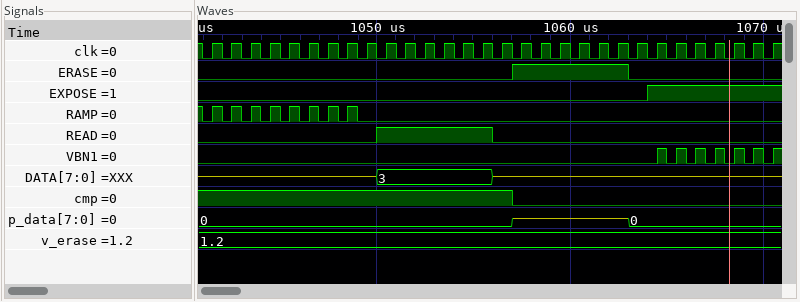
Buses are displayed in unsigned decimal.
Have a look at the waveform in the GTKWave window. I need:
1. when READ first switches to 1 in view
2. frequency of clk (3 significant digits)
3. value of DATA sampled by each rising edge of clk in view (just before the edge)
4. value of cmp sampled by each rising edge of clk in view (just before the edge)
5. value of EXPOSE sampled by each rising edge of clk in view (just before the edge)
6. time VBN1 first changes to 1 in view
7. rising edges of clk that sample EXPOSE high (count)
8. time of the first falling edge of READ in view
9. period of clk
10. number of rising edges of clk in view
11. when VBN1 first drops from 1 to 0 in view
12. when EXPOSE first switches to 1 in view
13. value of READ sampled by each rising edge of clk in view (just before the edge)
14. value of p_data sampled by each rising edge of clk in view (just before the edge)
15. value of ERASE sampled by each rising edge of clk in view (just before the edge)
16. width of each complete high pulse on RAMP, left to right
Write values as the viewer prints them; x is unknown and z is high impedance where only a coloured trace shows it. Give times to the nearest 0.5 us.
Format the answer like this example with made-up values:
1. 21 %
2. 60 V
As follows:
1. 1050 us
2. 1.00 MHz
3. z, z, z, z, z, z, z, z, z, 3, 3, 3, 3, 3, 3, z, z, z, z, z, z, z, z, z, z, z, z, z, z, z
4. 1 1 1 1 1 1 1 1 1 1 1 1 1 1 1 1 0 0 0 0 0 0 0 0 0 0 0 0 0 0
5. 0 0 0 0 0 0 0 0 0 0 0 0 0 0 0 0 0 0 0 0 0 0 0 1 1 1 1 1 1 1
6. 1064.5 us
7. 7
8. 1056 us
9. 1 us
10. 30
11. 1065 us
12. 1064 us
13. 0 0 0 0 0 0 0 0 0 1 1 1 1 1 1 0 0 0 0 0 0 0 0 0 0 0 0 0 0 0
14. 0, 0, 0, 0, 0, 0, 0, 0, 0, 0, 0, 0, 0, 0, 0, 0, z, z, z, z, z, z, 0, 0, 0, 0, 0, 0, 0, 0
15. 0 0 0 0 0 0 0 0 0 0 0 0 0 0 0 0 1 1 1 1 1 1 0 0 0 0 0 0 0 0
16. 0.5 us, 0.5 us, 0.5 us, 0.5 us, 0.5 us, 0.5 us, 0.5 us, 0.5 us
